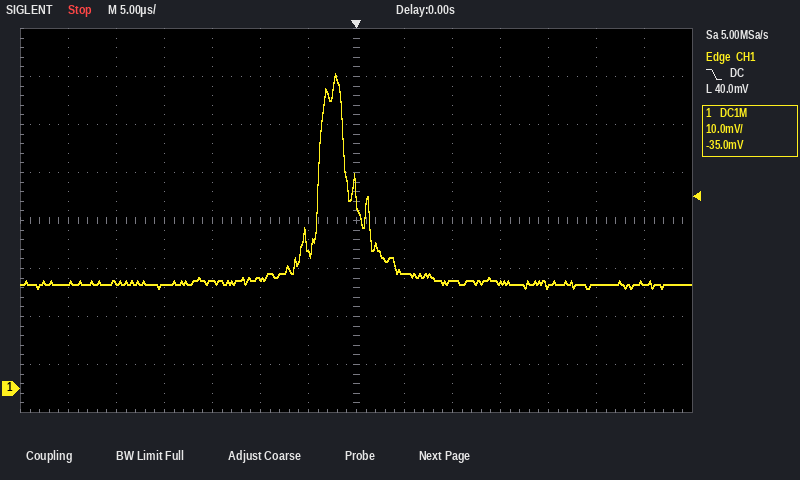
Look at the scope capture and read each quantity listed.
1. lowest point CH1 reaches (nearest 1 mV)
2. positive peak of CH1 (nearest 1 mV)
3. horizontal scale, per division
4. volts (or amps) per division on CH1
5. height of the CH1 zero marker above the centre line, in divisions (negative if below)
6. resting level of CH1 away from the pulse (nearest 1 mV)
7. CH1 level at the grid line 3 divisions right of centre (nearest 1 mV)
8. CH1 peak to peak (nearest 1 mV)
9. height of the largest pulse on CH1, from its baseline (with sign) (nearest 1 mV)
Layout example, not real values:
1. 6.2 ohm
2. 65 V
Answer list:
1. 21 mV
2. 66 mV
3. 5 µs
4. 10 mV
5. -3.5 div
6. 22 mV
7. 22 mV
8. 45 mV
9. +44 mV
